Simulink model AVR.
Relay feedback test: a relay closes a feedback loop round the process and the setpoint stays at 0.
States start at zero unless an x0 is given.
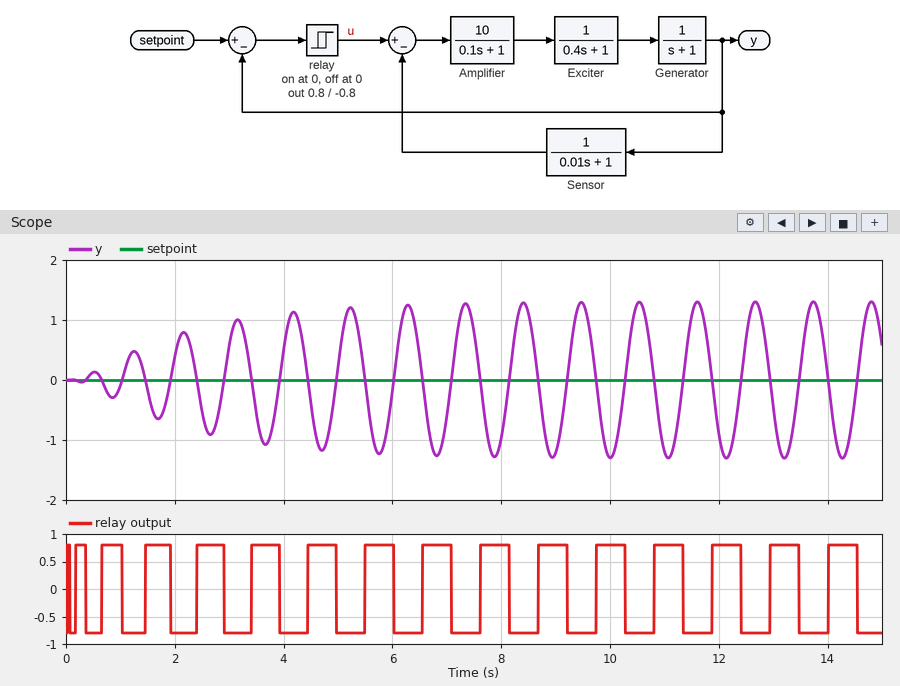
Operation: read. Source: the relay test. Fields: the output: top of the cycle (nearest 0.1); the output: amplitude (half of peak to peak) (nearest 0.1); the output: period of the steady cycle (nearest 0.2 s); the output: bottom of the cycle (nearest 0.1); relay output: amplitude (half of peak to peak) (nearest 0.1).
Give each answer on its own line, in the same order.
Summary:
1.3
1.3
1.0 s
-1.3
0.8
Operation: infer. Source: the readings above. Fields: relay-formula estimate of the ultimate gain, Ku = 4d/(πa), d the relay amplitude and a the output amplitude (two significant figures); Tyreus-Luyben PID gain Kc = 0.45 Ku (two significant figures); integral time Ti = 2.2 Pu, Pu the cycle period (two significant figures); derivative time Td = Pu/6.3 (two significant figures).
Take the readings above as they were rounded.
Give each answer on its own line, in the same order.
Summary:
0.78
0.35
2.2 s
0.16 s
